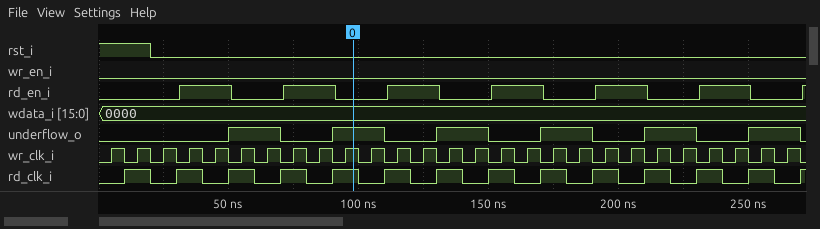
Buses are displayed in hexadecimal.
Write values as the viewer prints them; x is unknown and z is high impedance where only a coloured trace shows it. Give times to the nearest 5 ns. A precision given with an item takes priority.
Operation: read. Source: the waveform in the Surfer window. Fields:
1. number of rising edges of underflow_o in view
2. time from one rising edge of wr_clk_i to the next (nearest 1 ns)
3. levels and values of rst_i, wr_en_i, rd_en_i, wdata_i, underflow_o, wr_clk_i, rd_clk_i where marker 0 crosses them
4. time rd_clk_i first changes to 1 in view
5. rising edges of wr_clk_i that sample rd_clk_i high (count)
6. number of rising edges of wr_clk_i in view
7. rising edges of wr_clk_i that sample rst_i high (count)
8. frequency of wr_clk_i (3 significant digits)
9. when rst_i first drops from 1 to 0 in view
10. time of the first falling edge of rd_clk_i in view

6
10 ns
rst_i=0, wr_en_i=0, rd_en_i=0, wdata_i=0000, underflow_o=1, wr_clk_i=1, rd_clk_i=1
10 ns
13
27
2
100 MHz
20 ns
20 ns
